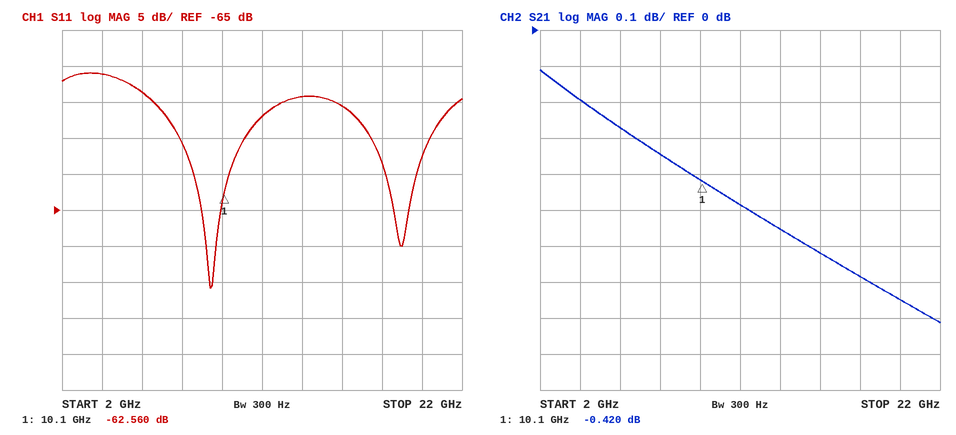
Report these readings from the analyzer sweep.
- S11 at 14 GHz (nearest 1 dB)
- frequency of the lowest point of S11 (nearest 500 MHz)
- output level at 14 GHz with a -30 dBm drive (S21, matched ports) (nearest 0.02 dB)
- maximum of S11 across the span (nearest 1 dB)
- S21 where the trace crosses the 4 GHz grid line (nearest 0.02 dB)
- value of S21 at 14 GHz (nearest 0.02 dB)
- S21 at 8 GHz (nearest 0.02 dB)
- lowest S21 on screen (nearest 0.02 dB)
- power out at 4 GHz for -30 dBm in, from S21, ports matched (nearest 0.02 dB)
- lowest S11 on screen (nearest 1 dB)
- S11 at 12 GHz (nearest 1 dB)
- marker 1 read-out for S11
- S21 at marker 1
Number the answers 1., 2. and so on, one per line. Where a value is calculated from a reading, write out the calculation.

1. -49 dB
2. 9.5 GHz
3. -30 dBm + (-0.56 dB) = -30.56 dBm
4. -46 dB
5. -0.20 dB
6. -0.56 dB
7. -0.34 dB
8. -0.82 dB
9. -30 dBm + (-0.20 dB) = -30.20 dBm
10. -76 dB
11. -52 dB
12. -62.560 dB
13. -0.420 dB
